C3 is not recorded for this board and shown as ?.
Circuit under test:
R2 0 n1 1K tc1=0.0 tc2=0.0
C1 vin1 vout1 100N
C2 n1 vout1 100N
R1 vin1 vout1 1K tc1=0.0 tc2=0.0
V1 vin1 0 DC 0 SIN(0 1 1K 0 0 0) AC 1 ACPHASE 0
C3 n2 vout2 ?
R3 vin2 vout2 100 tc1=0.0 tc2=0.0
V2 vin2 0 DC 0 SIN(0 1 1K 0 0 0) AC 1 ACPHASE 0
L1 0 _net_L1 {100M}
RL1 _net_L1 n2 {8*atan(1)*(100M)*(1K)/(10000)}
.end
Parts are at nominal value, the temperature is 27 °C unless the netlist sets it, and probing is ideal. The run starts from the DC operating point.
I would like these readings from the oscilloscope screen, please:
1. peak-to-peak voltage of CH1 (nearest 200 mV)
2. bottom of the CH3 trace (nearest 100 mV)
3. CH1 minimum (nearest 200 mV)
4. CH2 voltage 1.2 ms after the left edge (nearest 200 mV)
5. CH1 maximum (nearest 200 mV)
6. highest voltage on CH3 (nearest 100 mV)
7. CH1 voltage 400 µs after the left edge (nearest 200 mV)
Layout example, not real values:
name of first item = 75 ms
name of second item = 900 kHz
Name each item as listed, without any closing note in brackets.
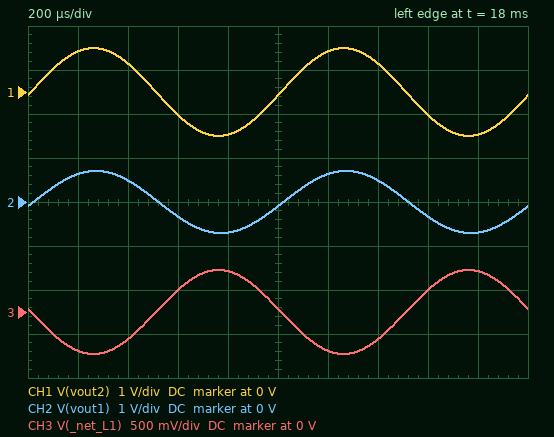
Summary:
peak-to-peak voltage of CH1 = 2.0 V
bottom of the CH3 trace = -500 mV
CH1 minimum = -1.0 V
CH2 voltage 1.2 ms after the left edge = 600 mV
CH1 maximum = 1.0 V
highest voltage on CH3 = 500 mV
CH1 voltage 400 µs after the left edge = 600 mV
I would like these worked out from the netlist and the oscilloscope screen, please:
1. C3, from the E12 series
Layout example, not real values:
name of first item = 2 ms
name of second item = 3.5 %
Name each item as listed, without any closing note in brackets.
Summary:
C3, from the E12 series = 82 nF
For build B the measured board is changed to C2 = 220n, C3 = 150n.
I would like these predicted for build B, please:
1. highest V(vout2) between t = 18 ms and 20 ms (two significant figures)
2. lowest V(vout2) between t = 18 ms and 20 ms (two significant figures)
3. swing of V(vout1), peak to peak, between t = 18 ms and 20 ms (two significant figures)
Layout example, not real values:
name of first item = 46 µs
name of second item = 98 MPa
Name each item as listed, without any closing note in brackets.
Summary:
highest V(vout2) between t = 18 ms and 20 ms = 970 mV
lowest V(vout2) between t = 18 ms and 20 ms = -970 mV
swing of V(vout1), peak to peak, between t = 18 ms and 20 ms = 1.2 V
